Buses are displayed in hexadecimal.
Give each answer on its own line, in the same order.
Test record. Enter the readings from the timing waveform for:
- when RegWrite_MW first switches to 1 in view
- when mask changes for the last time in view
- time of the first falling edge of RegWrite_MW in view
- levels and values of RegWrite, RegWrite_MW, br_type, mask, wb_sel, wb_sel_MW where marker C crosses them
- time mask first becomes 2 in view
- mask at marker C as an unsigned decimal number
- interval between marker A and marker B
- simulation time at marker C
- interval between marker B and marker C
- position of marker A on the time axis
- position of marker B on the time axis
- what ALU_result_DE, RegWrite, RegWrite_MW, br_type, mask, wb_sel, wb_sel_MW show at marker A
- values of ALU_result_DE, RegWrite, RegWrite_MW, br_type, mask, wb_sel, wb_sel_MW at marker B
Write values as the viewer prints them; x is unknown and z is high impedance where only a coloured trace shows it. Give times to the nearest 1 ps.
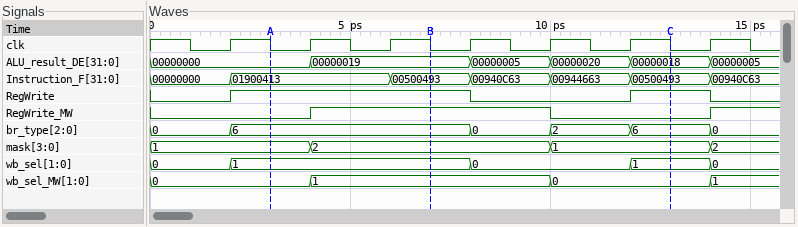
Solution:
4 ps
14 ps
10 ps
RegWrite=1, RegWrite_MW=0, br_type=6, mask=1, wb_sel=1, wb_sel_MW=0
4 ps
1
4 ps
13 ps
6 ps
3 ps
7 ps
ALU_result_DE=00000000, RegWrite=1, RegWrite_MW=0, br_type=6, mask=1, wb_sel=1, wb_sel_MW=0
ALU_result_DE=00000019, RegWrite=1, RegWrite_MW=1, br_type=6, mask=2, wb_sel=1, wb_sel_MW=1
